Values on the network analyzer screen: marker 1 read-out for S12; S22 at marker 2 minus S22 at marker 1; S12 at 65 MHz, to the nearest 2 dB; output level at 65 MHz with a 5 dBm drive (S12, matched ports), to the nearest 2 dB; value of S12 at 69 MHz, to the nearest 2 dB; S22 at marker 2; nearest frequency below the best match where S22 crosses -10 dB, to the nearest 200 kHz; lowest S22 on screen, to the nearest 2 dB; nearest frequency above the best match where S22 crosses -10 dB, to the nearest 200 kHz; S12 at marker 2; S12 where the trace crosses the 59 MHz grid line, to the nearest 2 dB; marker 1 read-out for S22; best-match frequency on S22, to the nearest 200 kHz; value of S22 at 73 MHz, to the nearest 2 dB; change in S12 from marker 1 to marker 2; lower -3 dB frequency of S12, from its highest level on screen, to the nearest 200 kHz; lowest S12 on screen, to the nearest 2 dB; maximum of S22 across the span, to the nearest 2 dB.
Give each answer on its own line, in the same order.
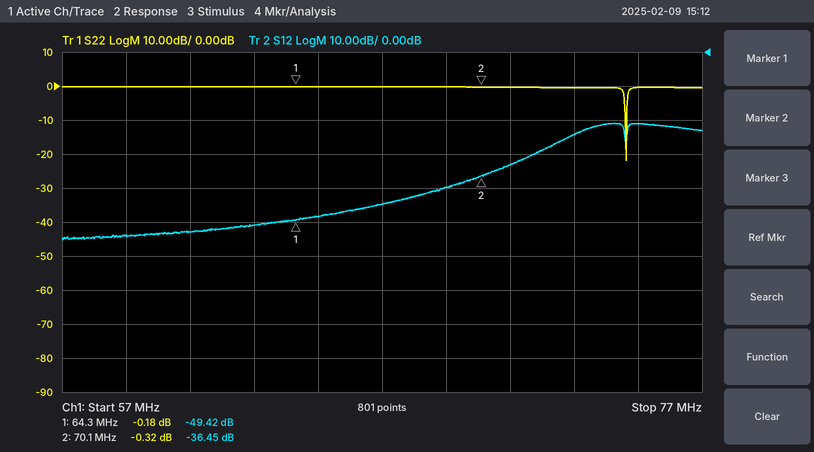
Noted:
-49.42 dB
-0.14 dB
-48 dB
-44 dBm
-40 dB
-0.32 dB
74.6 MHz
-22 dB
74.6 MHz
-36.45 dB
-54 dB
-0.18 dB
74.6 MHz
0 dB
12.97 dB
73.0 MHz
-56 dB
0 dB
